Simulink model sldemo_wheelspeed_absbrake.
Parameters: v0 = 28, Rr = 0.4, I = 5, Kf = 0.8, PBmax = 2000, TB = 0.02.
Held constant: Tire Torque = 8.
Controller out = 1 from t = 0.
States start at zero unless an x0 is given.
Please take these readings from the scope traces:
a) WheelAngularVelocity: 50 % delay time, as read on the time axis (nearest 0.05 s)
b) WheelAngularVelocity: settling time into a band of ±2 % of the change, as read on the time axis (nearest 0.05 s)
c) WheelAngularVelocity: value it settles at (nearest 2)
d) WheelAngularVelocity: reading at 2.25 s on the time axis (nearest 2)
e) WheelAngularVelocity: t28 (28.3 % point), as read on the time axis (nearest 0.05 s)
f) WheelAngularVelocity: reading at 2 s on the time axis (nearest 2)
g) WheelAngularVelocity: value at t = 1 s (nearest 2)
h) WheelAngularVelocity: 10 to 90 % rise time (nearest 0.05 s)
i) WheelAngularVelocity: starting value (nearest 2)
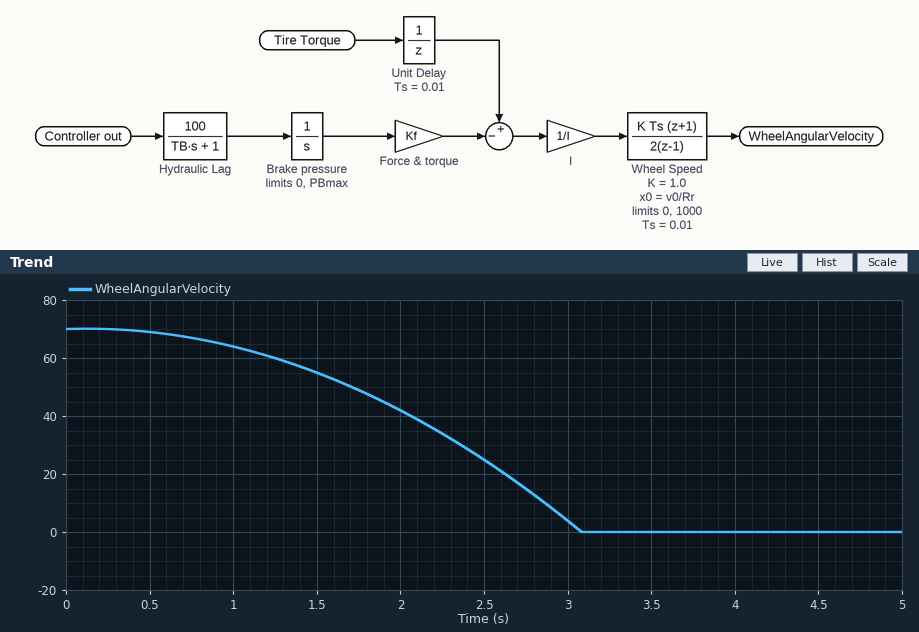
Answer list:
2.20 s
3.05 s
0
34
1.70 s
42
64
1.85 s
70
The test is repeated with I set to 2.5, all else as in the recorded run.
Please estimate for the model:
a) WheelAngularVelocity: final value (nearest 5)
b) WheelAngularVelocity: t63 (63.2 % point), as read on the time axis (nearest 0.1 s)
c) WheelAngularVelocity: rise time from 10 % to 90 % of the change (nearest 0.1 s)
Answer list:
0
1.8 s
1.3 s
